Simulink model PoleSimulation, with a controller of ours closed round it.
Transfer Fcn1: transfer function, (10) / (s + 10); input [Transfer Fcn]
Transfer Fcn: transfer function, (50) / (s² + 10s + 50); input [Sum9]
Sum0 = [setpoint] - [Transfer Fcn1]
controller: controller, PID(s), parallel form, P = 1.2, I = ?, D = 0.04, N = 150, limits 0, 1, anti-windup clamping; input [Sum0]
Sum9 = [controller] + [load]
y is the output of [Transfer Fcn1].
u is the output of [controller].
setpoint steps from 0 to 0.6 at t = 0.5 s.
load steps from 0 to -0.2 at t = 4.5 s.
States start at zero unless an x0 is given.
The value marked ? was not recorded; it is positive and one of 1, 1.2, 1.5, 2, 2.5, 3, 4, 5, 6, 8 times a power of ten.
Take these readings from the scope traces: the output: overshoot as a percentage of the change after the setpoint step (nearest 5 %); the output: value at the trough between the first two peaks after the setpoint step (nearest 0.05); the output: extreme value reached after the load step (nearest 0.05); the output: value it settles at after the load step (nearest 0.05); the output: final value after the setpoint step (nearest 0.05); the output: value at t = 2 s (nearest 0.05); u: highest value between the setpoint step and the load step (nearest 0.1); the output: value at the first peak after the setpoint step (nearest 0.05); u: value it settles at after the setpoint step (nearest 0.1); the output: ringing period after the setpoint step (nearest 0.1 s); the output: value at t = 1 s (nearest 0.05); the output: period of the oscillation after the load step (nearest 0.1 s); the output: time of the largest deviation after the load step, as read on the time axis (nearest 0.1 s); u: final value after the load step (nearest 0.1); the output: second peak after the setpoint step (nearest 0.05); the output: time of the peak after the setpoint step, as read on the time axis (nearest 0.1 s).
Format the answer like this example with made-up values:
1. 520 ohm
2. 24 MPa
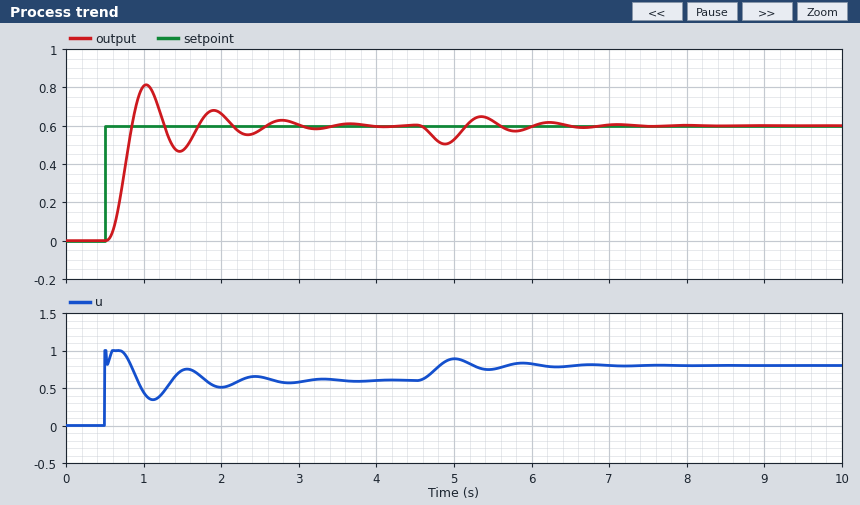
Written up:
1. 35 %
2. 0.45
3. 0.50
4. 0.60
5. 0.60
6. 0.65
7. 1.0
8. 0.80
9. 0.6
10. 0.9 s
11. 0.80
12. 0.9 s
13. 4.9 s
14. 0.8
15. 0.70
16. 1.0 s
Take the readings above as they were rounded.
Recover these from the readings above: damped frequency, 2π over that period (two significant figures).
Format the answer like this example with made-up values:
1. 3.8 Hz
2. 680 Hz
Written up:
1. 7.0 rad/s
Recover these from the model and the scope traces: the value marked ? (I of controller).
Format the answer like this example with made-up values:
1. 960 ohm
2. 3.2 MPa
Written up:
1. 8
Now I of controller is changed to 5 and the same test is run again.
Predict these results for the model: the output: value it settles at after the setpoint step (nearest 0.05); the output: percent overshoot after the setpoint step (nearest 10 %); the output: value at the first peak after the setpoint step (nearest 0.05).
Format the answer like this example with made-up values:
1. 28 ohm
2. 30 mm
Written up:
1. 0.60
2. 20 %
3. 0.70
